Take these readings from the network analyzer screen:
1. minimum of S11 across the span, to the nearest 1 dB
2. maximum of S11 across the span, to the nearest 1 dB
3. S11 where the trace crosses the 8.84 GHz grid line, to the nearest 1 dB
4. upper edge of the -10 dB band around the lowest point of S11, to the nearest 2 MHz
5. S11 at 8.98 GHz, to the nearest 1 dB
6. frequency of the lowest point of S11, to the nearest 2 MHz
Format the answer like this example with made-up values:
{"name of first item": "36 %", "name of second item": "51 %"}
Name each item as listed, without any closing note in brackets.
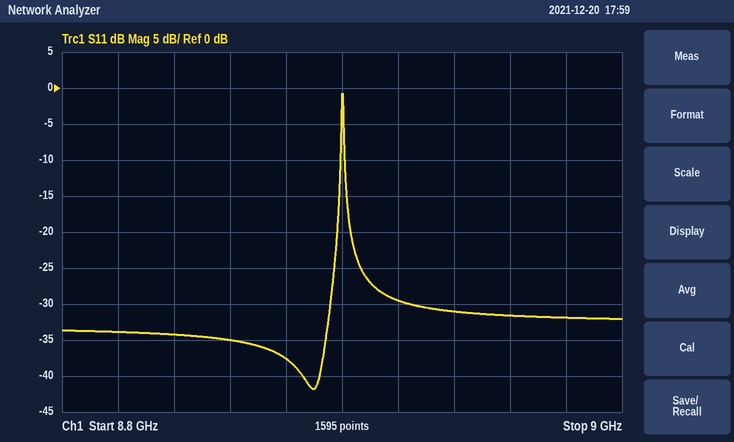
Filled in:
{"minimum of S11 across the span, to the nearest 1 dB": "-42 dB", "maximum of S11 across the span, to the nearest 1 dB": "-1 dB", "S11 where the trace crosses the 8.84 GHz grid line, to the nearest 1 dB": "-34 dB", "upper edge of the -10 dB band around the lowest point of S11, to the nearest 2 MHz": "8.900 GHz", "S11 at 8.98 GHz, to the nearest 1 dB": "-32 dB", "frequency of the lowest point of S11, to the nearest 2 MHz": "8.890 GHz"}
